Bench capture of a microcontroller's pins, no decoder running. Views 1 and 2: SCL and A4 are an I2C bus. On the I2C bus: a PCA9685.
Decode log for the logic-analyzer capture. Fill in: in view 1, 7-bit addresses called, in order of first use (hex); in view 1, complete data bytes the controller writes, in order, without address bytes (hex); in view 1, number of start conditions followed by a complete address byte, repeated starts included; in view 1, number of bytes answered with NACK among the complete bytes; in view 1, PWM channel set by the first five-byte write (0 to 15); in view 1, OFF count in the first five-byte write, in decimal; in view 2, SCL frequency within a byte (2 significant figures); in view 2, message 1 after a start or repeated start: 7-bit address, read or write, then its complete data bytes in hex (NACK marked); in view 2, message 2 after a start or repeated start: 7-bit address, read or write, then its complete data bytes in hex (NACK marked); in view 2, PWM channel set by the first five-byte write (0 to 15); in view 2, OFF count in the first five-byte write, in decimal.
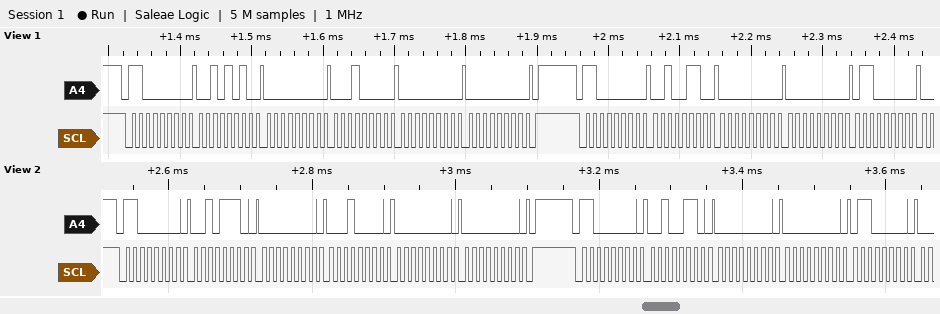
0x60
2A 00 10 00 00 26 00 00 60
2
0
9
0
100 kHz
0x60 write: 2E 00 10 00 00
0x60 write: 26 00 00 60
10
0
